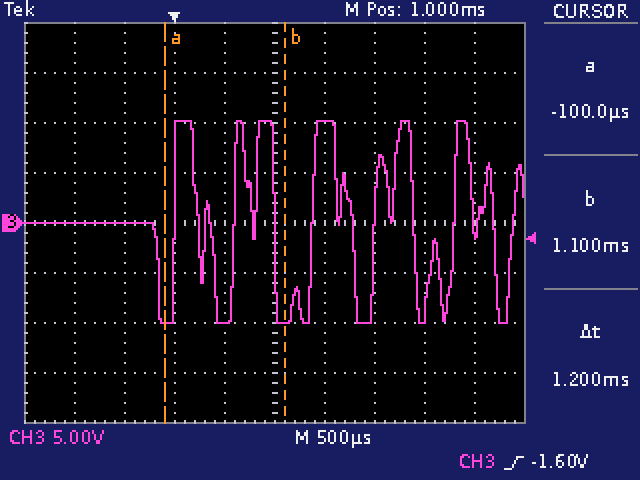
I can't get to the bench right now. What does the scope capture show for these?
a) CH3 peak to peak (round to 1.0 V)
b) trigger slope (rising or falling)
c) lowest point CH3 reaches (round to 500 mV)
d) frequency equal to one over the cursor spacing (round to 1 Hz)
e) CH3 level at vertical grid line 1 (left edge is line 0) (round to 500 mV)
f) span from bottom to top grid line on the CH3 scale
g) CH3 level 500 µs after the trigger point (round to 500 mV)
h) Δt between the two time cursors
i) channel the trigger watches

20.0 V
rising
-10.0 V
833 Hz
0.0 V
40 V
-10.0 V
1.2 ms
CH3
